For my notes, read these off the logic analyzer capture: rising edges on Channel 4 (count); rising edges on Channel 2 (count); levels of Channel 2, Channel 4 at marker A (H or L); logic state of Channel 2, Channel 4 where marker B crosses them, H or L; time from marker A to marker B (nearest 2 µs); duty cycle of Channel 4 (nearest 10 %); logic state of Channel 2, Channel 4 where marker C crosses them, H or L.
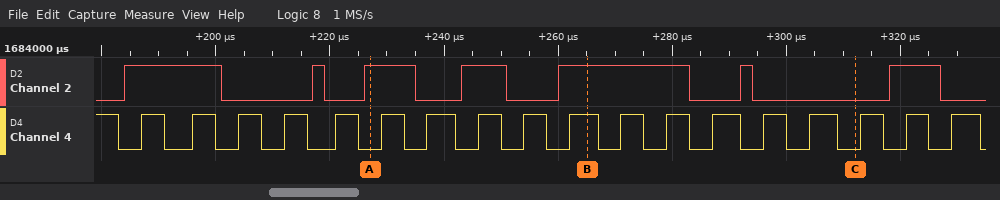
18
7
Channel 2=H, Channel 4=L
Channel 2=H, Channel 4=H
38 µs
50 %
Channel 2=L, Channel 4=L
